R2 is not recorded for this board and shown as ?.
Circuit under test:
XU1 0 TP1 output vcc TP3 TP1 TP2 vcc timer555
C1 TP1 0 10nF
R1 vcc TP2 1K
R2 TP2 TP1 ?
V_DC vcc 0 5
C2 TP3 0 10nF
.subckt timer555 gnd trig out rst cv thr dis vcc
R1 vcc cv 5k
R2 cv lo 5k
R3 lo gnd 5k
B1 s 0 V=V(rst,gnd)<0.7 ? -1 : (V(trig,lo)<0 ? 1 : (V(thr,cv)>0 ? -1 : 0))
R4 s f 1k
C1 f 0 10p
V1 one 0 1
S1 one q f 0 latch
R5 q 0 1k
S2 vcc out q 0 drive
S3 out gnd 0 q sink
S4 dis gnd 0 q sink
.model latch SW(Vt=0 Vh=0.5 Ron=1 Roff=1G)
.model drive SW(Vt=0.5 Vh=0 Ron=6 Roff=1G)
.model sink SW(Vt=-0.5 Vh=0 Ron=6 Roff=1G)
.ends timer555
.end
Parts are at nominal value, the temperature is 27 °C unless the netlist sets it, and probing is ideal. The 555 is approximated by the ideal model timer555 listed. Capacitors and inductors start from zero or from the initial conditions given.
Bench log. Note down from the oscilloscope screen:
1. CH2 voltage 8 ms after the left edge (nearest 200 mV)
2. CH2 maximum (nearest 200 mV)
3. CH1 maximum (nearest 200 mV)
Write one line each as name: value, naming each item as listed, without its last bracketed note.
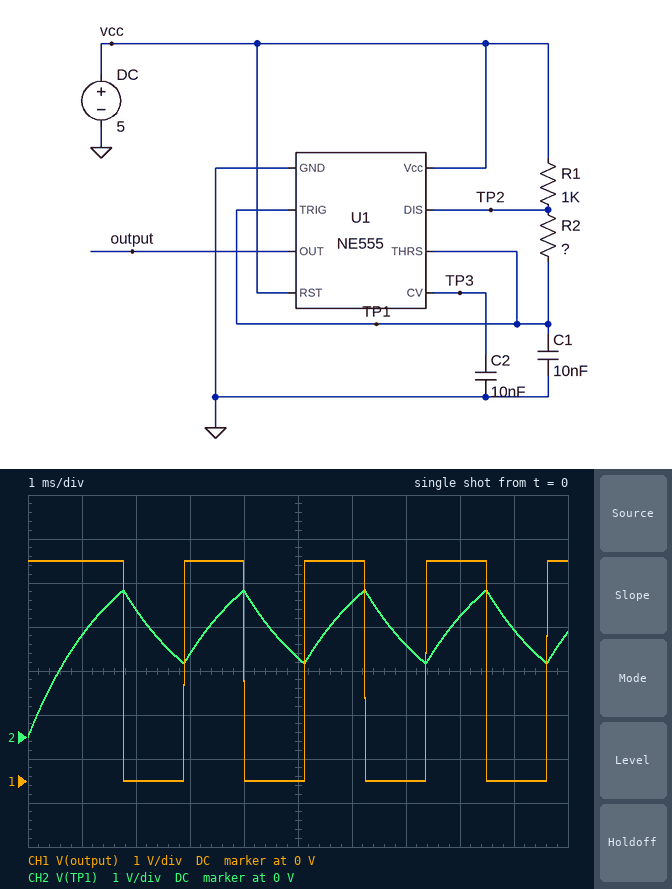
CH2 voltage 8 ms after the left edge: 2.8 V
CH2 maximum: 3.4 V
CH1 maximum: 5.0 V
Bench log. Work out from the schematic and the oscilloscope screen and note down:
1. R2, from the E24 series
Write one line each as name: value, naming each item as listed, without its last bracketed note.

R2, from the E24 series: 160 kΩ
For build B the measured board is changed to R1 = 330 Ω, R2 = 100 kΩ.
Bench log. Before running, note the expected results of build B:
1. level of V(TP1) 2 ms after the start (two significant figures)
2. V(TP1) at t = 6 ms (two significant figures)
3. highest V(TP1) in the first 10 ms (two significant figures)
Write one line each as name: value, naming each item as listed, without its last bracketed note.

level of V(TP1) 2 ms after the start: 2.2 V
V(TP1) at t = 6 ms: 1.8 V
highest V(TP1) in the first 10 ms: 3.3 V
